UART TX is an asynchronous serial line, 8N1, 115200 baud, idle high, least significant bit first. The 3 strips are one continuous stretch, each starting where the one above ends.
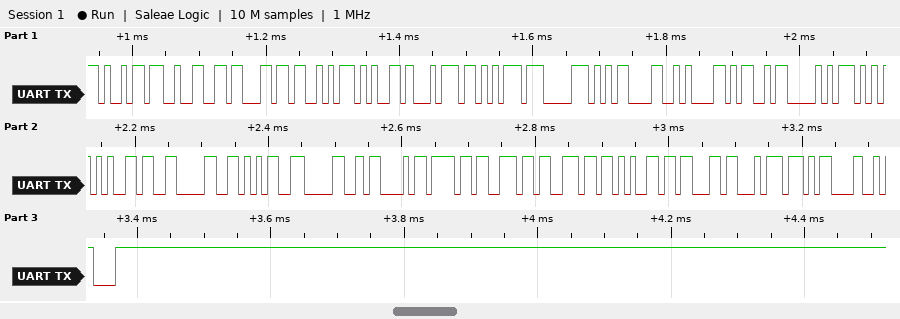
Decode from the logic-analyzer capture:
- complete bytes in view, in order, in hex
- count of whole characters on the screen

69 32 63 53 65 74 75 70 0D 0A 4D 50 55 36 30 35 30 43 6F 6E 6E 65 63 74 0D 0A
26
